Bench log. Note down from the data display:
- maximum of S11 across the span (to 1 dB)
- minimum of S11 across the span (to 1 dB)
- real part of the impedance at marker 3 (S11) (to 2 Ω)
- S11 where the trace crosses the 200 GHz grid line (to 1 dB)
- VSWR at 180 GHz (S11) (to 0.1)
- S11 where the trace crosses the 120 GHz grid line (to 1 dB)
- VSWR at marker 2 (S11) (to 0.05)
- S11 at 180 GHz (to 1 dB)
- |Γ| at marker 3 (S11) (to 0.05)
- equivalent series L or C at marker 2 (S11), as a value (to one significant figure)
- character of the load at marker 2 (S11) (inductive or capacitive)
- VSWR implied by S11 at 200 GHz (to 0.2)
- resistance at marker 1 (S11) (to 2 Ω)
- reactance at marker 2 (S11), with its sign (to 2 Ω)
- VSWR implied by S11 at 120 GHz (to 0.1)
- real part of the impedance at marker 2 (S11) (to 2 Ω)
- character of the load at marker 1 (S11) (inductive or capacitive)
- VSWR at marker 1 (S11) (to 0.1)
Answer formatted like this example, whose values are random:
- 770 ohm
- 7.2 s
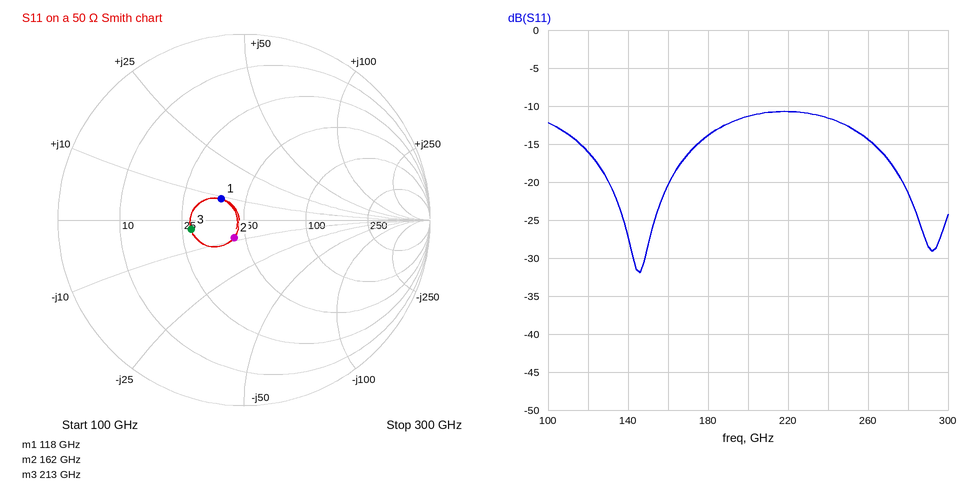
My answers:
- -11 dB
- -32 dB
- 28 Ω
- -11 dB
- 1.5
- -16 dB
- 1.25
- -14 dB
- 0.30
- 100 fF
- capacitive
- 1.8
- 38 Ω
- -8 Ω
- 1.4
- 44 Ω
- inductive
- 1.4
